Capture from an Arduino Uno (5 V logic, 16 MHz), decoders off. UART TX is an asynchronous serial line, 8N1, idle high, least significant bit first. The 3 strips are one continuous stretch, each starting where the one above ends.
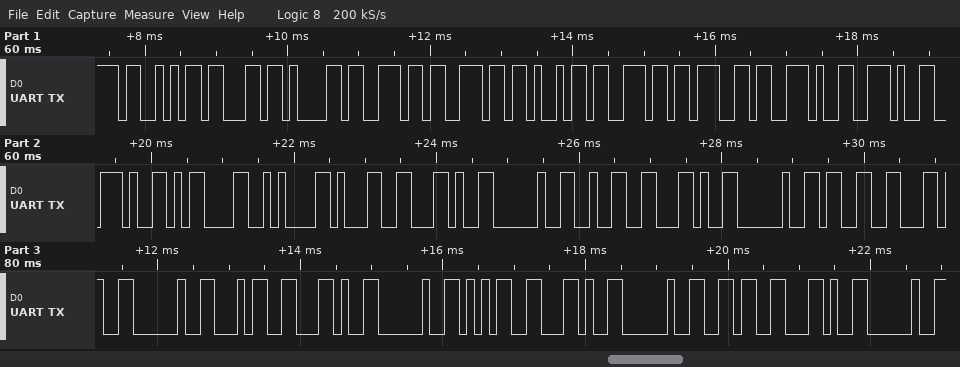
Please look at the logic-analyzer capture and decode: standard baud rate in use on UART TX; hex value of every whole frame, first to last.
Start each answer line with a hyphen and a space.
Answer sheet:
- 9600 baud
- 53 63 61 6E 6E 69 6E 67 2E 2E 2E 0D 0A 31 2C 20 32 2C 20 33 2C 20 34 2C 20 35 2C 20 36 2C 20
